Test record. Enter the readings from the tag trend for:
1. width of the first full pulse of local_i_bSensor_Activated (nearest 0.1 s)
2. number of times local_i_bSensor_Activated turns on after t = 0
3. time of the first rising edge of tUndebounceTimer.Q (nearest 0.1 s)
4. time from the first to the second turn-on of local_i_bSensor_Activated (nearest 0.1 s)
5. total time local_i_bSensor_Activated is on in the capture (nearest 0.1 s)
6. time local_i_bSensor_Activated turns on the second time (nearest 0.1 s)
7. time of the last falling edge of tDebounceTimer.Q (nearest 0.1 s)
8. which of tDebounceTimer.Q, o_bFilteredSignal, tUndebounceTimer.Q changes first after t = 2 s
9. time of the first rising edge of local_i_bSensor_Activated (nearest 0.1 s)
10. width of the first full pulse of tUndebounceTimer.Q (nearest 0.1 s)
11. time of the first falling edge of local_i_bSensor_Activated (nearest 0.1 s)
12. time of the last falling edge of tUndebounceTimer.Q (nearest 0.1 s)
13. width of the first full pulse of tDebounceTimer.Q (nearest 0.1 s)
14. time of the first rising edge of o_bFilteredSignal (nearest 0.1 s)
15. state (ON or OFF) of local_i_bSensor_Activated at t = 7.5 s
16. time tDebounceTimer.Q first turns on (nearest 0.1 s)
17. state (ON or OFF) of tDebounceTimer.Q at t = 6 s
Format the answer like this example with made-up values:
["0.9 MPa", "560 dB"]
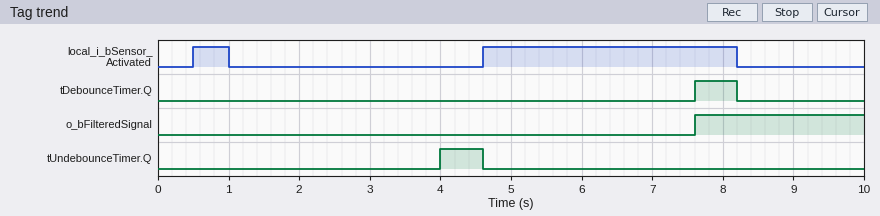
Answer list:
["0.5 s", "2", "4.0 s", "4.1 s", "4.1 s", "4.6 s", "8.2 s", "tUndebounceTimer.Q", "0.5 s", "0.6 s", "1.0 s", "4.6 s", "0.6 s", "7.6 s", "ON", "7.6 s", "OFF"]
